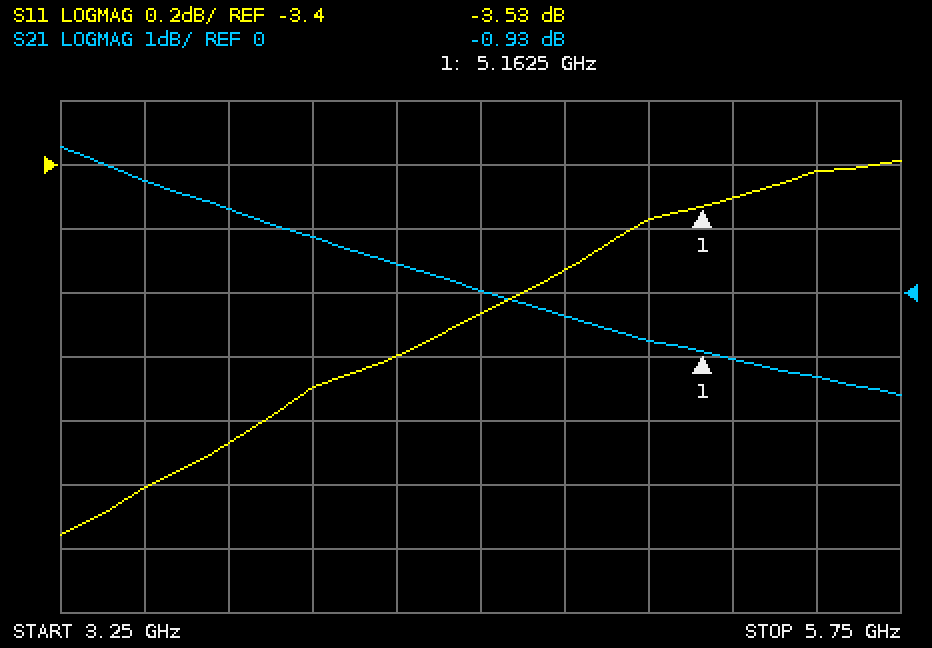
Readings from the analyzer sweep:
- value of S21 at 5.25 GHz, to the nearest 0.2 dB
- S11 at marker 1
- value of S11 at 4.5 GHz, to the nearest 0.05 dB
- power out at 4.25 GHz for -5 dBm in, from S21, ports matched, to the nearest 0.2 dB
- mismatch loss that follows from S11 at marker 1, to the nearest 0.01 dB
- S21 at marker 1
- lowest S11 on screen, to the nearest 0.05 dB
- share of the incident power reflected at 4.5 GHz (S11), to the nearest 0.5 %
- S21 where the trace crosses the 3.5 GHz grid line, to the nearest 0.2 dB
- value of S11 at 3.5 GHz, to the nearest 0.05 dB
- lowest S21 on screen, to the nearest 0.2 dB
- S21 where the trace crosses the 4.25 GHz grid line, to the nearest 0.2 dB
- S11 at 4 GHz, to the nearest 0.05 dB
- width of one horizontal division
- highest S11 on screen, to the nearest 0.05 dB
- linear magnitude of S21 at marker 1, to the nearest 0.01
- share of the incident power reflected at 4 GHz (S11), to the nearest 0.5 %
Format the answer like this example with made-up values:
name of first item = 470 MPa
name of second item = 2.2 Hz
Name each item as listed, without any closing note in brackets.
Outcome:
value of S21 at 5.25 GHz, to the nearest 0.2 dB = -1.0 dB
S11 at marker 1 = -3.53 dB
value of S11 at 4.5 GHz, to the nearest 0.05 dB = -3.85 dB
power out at 4.25 GHz for -5 dBm in, from S21, ports matched, to the nearest 0.2 dB = -4.6 dBm
mismatch loss that follows from S11 at marker 1, to the nearest 0.01 dB = 2.55 dB
S21 at marker 1 = -0.93 dB
lowest S11 on screen, to the nearest 0.05 dB = -4.55 dB
share of the incident power reflected at 4.5 GHz (S11), to the nearest 0.5 % = 41.0 %
S21 where the trace crosses the 3.5 GHz grid line, to the nearest 0.2 dB = 1.8 dB
value of S11 at 3.5 GHz, to the nearest 0.05 dB = -4.40 dB
lowest S21 on screen, to the nearest 0.2 dB = -1.6 dB
S21 where the trace crosses the 4.25 GHz grid line, to the nearest 0.2 dB = 0.4 dB
S11 at 4 GHz, to the nearest 0.05 dB = -4.10 dB
width of one horizontal division = 250 MHz
highest S11 on screen, to the nearest 0.05 dB = -3.40 dB
linear magnitude of S21 at marker 1, to the nearest 0.01 = 0.90
share of the incident power reflected at 4 GHz (S11), to the nearest 0.5 % = 39.0 %
